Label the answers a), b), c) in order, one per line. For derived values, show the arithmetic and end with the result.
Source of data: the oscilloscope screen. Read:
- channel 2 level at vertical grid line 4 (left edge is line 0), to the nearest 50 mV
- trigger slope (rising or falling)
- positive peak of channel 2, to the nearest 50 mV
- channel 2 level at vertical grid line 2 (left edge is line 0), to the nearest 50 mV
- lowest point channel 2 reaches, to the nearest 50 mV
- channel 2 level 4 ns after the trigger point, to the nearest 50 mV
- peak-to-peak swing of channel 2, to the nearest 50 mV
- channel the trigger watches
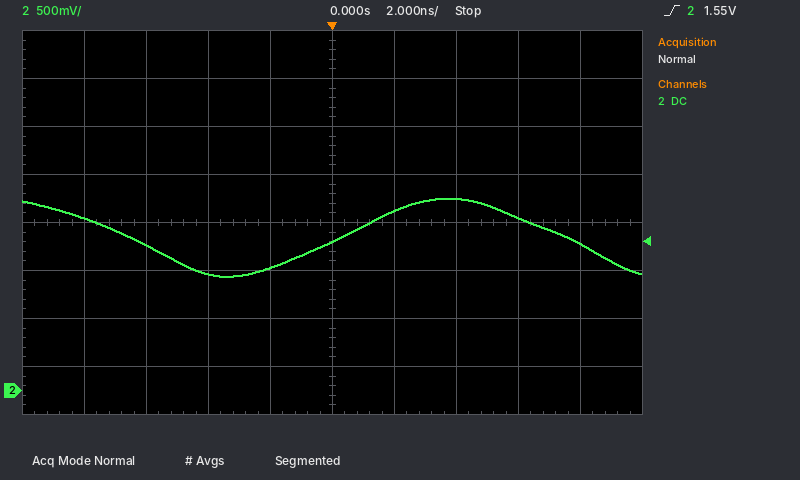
a) 1.30 V
b) rising
c) 2.00 V
d) 1.50 V
e) 1.20 V
f) 2.00 V
g) 2.00 V − (1.20 V) = 800 mV
h) channel 2
